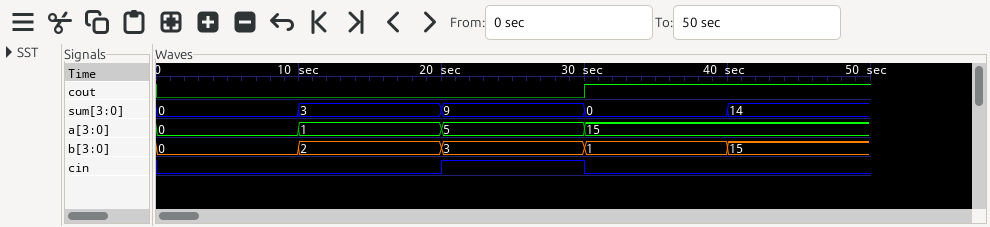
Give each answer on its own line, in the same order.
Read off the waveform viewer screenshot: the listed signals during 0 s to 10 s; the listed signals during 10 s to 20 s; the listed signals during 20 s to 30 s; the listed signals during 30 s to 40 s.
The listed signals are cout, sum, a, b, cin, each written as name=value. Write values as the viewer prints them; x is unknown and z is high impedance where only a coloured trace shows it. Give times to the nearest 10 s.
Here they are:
cout=0, sum=0, a=0, b=0, cin=0
cout=0, sum=3, a=1, b=2, cin=0
cout=0, sum=9, a=5, b=3, cin=1
cout=1, sum=0, a=15, b=1, cin=0
